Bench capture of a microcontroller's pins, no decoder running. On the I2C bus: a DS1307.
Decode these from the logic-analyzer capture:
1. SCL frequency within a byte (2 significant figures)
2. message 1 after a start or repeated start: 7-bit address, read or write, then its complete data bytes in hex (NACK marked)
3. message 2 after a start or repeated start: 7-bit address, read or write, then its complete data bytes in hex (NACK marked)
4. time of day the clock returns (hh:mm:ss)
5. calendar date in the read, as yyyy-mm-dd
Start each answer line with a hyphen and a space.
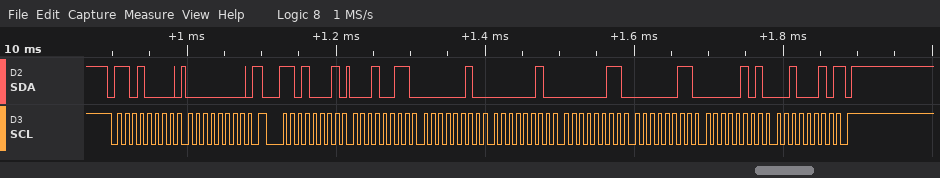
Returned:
- 100 kHz
- 0x68 write: 00
- 0x68 read: 13 02 02 03 03 05 22 NACK
- 02:02:13
- 2022-05-03
